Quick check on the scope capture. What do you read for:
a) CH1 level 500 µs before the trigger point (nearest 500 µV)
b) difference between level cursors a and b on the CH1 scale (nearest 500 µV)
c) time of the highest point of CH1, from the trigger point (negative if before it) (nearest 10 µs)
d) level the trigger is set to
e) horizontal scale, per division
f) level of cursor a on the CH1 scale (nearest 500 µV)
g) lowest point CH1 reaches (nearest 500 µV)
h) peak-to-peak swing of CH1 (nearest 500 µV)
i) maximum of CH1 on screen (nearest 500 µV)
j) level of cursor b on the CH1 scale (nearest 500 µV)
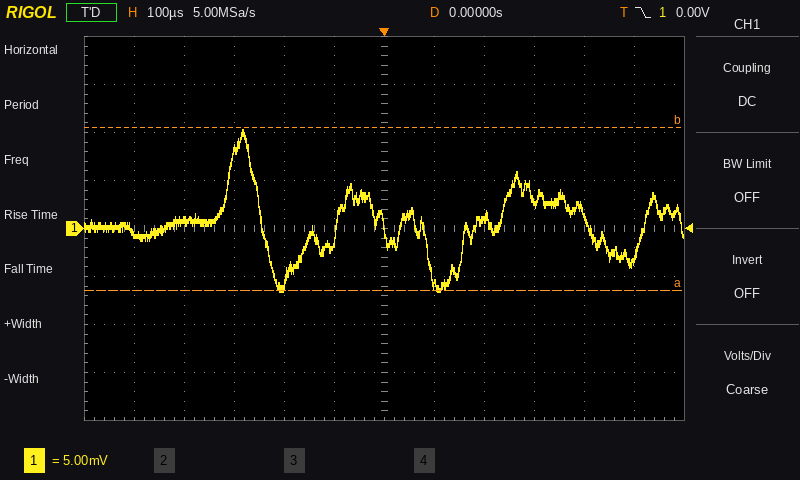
-500 µV
17.0 mV
-280 µs
0.00 V
100 µs
-6.5 mV
-6.5 mV
17.0 mV
10.5 mV
10.5 mV
